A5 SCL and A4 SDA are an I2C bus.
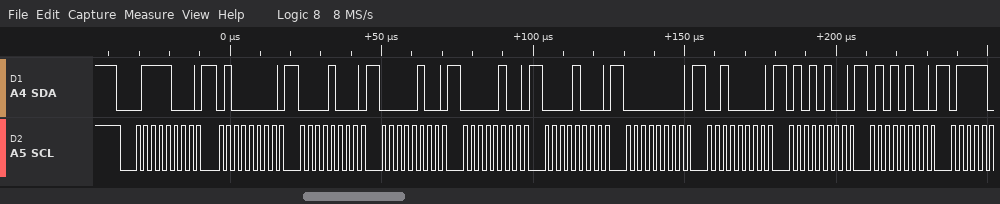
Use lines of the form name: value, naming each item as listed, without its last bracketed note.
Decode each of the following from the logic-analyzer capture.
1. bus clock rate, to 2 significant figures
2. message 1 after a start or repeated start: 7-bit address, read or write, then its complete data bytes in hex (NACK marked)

bus clock rate, to 2 significant figures: 400 kHz
message 1 after a start or repeated start: 7-bit address, read or write, then its complete data bytes in hex: 0x3C write: 40 08 04 04 08 00 20 54 54
